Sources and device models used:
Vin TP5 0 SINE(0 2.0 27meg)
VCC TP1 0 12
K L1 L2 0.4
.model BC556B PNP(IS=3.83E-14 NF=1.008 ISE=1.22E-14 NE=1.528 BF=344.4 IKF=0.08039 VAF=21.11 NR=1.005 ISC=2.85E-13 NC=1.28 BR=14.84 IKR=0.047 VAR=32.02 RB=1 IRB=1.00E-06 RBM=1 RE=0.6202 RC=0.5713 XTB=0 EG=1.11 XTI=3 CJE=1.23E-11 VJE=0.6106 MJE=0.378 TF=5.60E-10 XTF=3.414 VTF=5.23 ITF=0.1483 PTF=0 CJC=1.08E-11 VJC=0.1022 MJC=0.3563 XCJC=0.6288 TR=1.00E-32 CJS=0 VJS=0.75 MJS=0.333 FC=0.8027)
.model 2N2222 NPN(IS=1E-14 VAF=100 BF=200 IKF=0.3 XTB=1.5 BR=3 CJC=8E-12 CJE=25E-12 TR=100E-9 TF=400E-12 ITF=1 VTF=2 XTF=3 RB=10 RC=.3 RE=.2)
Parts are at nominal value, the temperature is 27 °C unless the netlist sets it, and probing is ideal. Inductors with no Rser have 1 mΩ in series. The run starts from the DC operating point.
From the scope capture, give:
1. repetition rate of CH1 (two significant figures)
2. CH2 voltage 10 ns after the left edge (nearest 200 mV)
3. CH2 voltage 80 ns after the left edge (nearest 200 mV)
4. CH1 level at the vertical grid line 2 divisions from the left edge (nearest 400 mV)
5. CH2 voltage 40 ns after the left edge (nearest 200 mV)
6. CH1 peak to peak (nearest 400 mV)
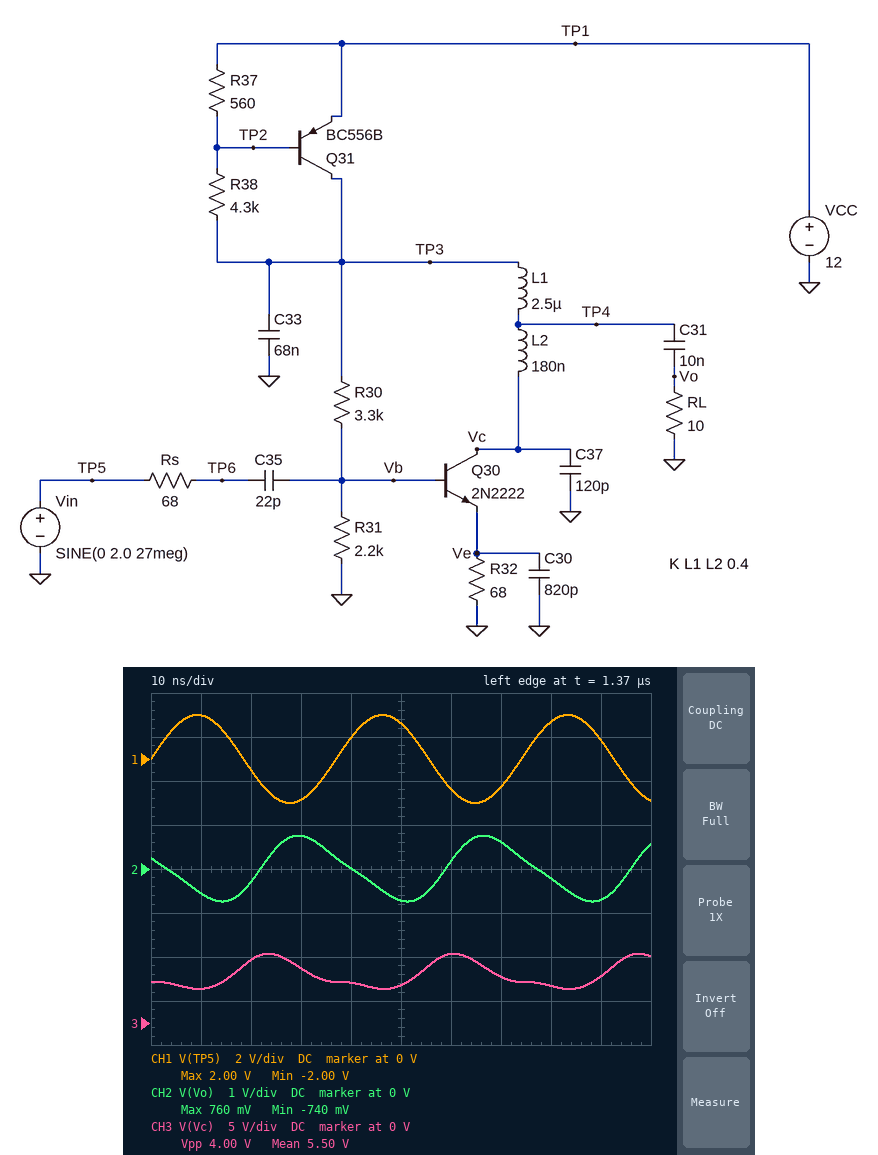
27 MHz
-600 mV
-200 mV
-400 mV
0 V
4.0 V
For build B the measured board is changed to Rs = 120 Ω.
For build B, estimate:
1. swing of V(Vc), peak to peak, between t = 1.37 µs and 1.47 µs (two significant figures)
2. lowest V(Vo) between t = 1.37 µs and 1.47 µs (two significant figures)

3.9 V
-720 mV
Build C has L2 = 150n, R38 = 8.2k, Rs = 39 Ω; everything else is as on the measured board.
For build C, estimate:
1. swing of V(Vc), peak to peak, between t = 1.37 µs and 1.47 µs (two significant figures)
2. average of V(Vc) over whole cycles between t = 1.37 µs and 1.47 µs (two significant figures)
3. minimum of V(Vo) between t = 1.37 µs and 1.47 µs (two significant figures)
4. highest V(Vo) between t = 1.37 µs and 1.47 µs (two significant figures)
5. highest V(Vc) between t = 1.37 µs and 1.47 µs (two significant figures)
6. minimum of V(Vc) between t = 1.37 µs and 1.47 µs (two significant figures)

1.5 V
2.0 V
-300 mV
270 mV
2.9 V
1.3 V
